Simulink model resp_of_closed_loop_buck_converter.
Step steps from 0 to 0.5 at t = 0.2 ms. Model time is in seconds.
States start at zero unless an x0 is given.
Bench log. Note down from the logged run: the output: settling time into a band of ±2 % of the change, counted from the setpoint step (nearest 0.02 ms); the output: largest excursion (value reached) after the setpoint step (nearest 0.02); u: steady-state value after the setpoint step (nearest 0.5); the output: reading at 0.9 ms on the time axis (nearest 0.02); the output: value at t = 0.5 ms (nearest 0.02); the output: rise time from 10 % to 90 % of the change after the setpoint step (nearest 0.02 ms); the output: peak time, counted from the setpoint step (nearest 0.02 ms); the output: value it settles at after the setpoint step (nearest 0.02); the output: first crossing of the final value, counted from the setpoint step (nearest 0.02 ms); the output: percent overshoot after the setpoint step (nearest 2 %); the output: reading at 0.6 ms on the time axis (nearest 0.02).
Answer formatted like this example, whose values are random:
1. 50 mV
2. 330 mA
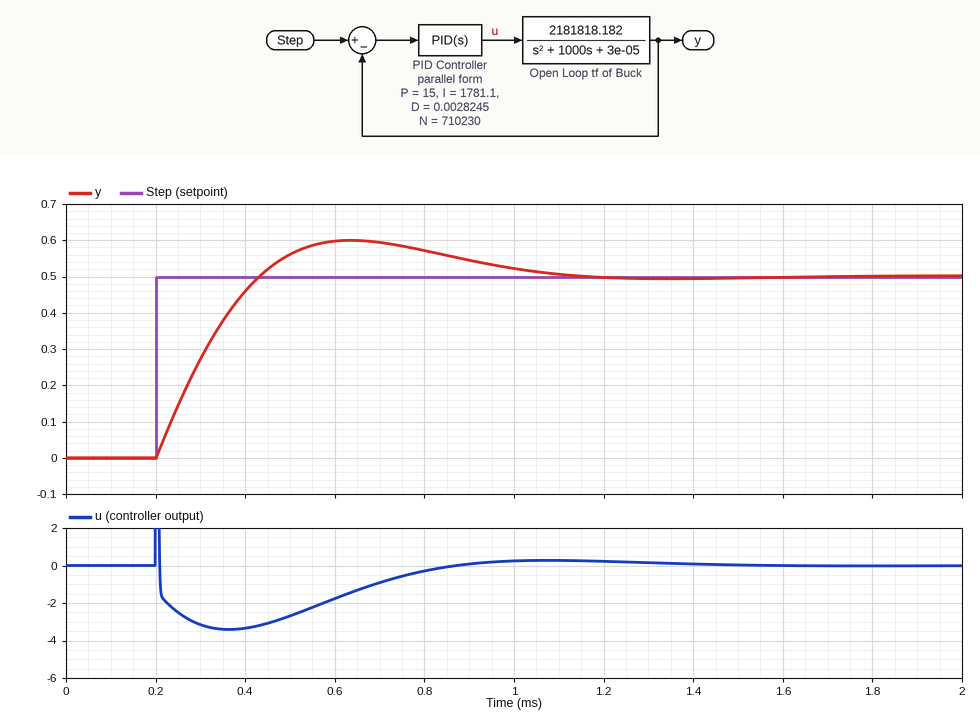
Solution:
1. 0.86 ms
2. 0.60
3. 0.0
4. 0.54
5. 0.56
6. 0.18 ms
7. 0.44 ms
8. 0.50
9. 0.24 ms
10. 20 %
11. 0.60
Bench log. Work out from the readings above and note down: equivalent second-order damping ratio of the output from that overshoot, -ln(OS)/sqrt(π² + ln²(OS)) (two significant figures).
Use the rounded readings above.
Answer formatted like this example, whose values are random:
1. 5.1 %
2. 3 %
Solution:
1. 0.46
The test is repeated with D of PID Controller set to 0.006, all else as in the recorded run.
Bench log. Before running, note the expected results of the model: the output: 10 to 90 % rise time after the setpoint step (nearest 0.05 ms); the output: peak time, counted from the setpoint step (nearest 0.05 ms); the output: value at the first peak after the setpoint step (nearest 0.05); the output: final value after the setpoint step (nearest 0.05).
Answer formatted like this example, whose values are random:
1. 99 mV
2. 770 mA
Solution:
1. 0.15 ms
2. 0.35 ms
3. 0.55
4. 0.50
